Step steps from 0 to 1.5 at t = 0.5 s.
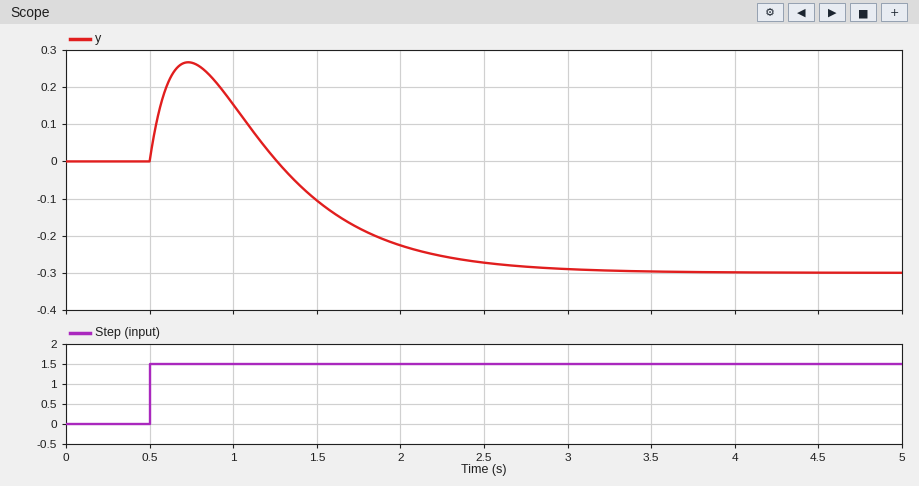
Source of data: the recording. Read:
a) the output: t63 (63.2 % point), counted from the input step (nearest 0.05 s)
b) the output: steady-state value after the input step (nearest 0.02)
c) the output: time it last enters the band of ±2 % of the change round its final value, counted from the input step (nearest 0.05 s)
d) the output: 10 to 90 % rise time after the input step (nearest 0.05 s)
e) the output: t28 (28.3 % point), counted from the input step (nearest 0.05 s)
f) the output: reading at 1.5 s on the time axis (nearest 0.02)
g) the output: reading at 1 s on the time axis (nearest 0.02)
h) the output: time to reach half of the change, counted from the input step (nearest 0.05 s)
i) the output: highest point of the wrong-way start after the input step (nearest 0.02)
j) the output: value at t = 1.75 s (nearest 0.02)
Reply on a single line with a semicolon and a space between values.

1.30 s; -0.30; 2.75 s; 1.15 s; 0.95 s; -0.10; 0.16; 1.15 s; 0.26; -0.18
